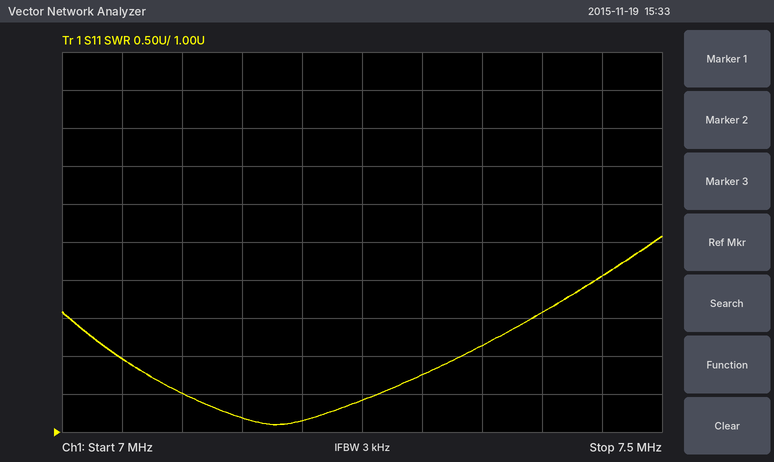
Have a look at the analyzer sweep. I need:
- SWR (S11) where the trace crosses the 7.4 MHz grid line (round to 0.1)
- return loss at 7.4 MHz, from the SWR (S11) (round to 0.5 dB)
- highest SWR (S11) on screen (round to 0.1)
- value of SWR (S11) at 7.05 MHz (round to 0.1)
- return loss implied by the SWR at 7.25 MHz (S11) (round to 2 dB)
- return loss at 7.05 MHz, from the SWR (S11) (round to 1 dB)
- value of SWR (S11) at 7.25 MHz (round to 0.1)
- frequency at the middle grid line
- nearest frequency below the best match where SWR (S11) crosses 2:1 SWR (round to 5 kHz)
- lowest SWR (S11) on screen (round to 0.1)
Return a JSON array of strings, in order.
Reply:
["2.6", "7.0 dB", "3.6", "2.0", "16 dB", "10 dB", "1.4", "7.25 MHz", "7.045 MHz", "1.1"]
